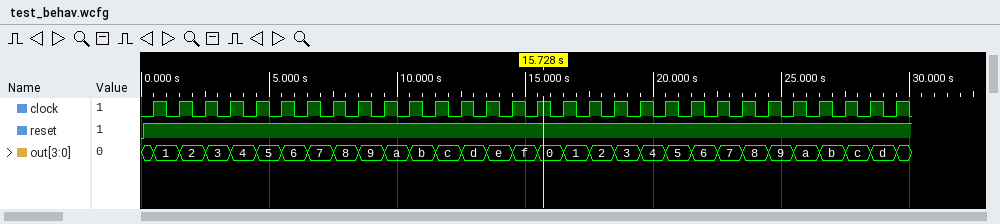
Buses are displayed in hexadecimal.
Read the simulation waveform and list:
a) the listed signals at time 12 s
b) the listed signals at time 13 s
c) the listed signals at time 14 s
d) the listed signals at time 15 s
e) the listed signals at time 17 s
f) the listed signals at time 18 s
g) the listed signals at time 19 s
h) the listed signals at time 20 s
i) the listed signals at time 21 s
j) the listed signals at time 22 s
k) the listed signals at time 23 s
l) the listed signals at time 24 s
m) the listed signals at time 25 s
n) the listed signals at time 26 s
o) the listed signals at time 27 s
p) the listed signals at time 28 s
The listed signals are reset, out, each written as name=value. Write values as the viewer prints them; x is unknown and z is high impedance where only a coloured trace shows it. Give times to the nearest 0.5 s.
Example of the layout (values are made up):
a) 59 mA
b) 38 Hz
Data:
a) reset=1, out=c
b) reset=1, out=d
c) reset=1, out=e
d) reset=1, out=f
e) reset=1, out=1
f) reset=1, out=2
g) reset=1, out=3
h) reset=1, out=4
i) reset=1, out=5
j) reset=1, out=6
k) reset=1, out=7
l) reset=1, out=8
m) reset=1, out=9
n) reset=1, out=a
o) reset=1, out=b
p) reset=1, out=c
